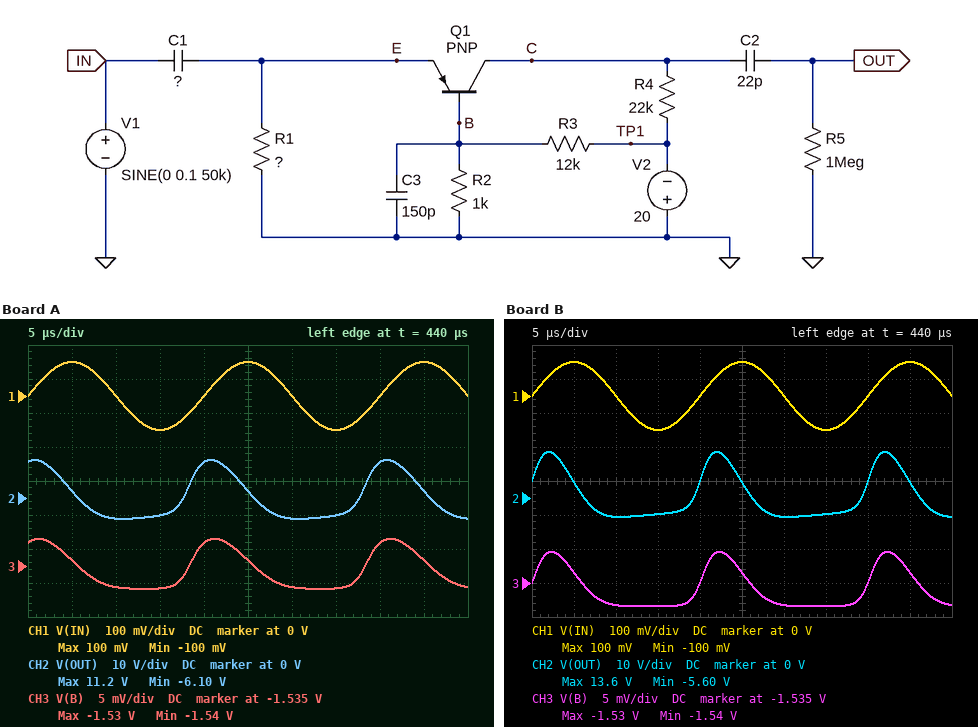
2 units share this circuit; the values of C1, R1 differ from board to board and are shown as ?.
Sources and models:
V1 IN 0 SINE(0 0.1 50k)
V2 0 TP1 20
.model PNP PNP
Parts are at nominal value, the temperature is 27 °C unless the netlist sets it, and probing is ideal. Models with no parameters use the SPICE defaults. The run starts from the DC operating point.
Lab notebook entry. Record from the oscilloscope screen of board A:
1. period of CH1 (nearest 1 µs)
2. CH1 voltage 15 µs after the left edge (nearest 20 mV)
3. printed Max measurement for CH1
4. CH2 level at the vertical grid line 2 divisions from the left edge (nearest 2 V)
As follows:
20 µs
-100 mV
100 mV
-6 V
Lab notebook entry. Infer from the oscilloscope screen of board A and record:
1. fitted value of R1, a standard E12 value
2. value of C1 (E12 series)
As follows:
2.7 kΩ
18 nF
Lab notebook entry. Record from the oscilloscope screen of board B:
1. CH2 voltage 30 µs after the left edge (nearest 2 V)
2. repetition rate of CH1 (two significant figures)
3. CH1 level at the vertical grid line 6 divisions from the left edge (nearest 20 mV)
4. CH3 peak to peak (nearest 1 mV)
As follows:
-6 V
50 kHz
0 V
8 mV
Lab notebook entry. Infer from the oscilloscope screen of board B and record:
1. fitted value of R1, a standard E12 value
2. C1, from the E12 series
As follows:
3.3 kΩ
27 nF
